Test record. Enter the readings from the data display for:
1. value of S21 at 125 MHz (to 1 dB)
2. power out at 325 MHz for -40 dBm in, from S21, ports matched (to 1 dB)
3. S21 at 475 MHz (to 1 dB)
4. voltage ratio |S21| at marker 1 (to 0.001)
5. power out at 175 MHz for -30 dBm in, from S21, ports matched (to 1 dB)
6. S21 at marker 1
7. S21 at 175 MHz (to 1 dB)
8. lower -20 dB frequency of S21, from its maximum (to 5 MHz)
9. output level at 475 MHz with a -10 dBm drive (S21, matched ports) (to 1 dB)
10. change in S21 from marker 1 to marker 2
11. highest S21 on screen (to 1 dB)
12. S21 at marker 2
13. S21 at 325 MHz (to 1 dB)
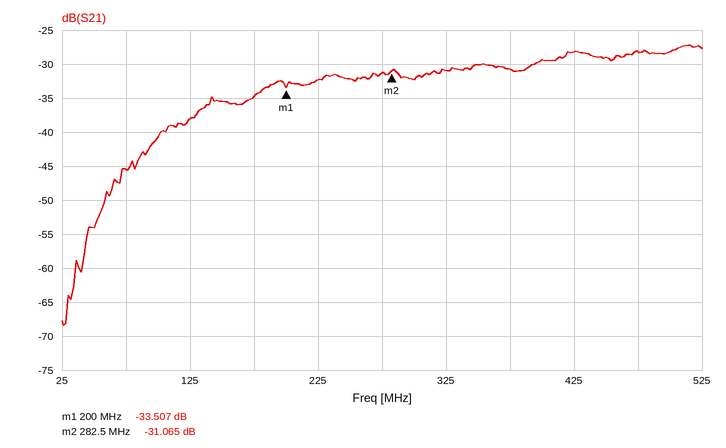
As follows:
-38 dB
-71 dBm
-28 dB
0.021
-65 dBm
-33.507 dB
-35 dB
70 MHz
-38 dBm
2.442 dB
-27 dB
-31.065 dB
-31 dB
